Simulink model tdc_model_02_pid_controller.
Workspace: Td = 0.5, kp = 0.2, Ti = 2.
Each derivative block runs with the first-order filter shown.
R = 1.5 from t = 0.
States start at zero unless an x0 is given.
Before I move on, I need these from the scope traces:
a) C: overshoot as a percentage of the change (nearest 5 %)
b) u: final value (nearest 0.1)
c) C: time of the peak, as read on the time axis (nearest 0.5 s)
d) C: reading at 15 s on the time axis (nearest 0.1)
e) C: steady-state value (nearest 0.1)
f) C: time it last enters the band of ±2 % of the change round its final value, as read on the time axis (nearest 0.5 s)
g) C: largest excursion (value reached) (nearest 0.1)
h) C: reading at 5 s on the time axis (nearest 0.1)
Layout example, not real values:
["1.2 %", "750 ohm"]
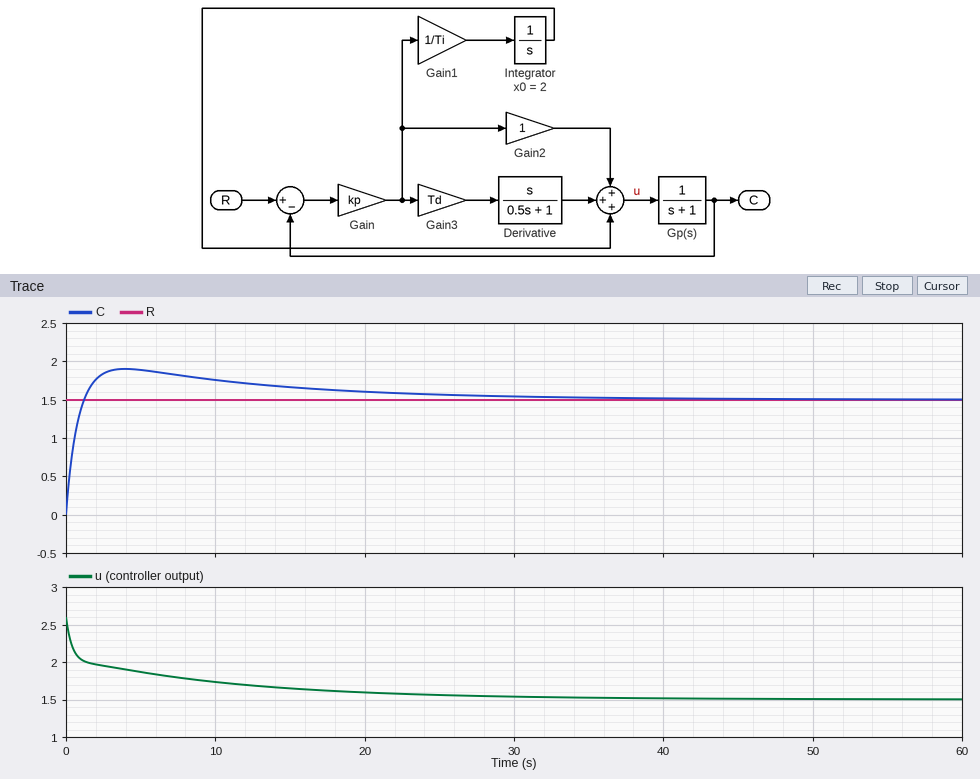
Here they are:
["25 %", "1.5", "4.0 s", "1.7", "1.5", "33.5 s", "1.9", "1.9"]
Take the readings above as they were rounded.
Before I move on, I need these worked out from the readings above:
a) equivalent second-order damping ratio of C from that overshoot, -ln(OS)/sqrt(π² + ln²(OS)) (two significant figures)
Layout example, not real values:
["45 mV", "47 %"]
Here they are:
["0.40"]
